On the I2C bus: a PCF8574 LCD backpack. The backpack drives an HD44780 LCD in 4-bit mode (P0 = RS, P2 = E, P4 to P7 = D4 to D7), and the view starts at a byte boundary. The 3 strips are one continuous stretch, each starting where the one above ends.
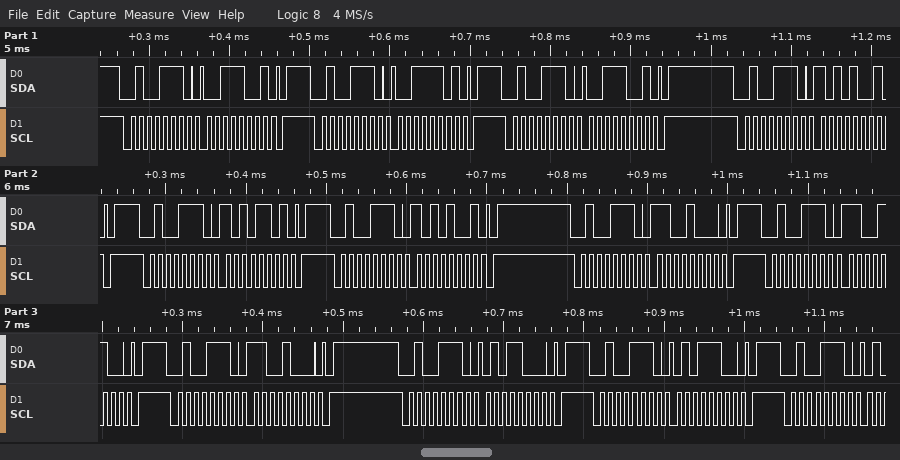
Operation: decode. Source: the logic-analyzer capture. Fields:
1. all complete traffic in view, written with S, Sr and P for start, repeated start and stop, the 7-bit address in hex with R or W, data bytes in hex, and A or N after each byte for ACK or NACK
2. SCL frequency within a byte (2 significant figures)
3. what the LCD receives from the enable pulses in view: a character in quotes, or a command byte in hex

S 27W A 39 A P S 27W A 3D A P S 27W A 39 A P S 27W A A9 A P S 27W A AD A P S 27W A A9 A P S 27W A C8 A P S 27W A CC A P S 27W A C8 A P S 27W A 58 A P S 27W A 5C A P S 27W A
100 kHz
':'
